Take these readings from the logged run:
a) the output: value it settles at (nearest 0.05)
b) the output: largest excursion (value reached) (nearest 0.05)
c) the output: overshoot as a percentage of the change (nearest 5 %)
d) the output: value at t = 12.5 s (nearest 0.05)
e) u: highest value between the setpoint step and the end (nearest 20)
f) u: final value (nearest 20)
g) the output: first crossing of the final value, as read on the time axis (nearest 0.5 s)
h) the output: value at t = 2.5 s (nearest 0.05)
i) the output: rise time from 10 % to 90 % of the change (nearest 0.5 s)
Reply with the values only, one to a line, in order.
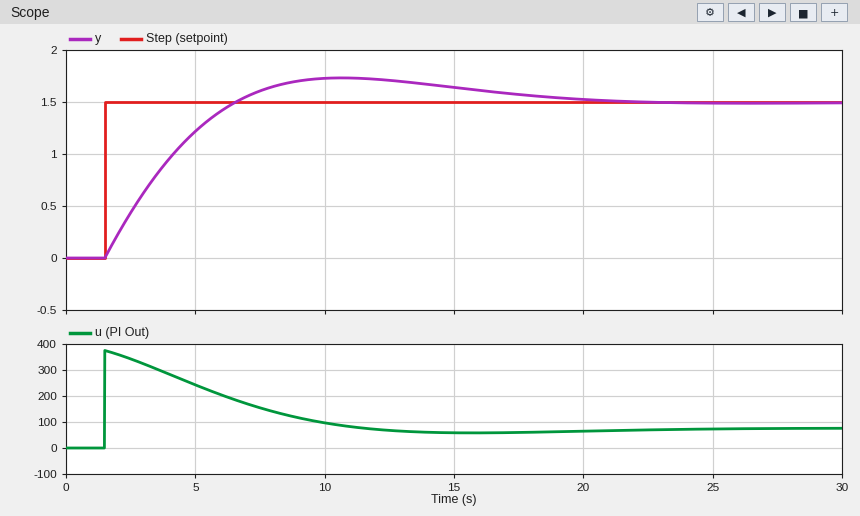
1.50
1.75
15 %
1.70
380
80
6.5 s
0.45
4.0 s
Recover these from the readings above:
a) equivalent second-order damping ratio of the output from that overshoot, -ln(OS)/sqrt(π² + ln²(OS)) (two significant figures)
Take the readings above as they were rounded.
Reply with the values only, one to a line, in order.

0.52
